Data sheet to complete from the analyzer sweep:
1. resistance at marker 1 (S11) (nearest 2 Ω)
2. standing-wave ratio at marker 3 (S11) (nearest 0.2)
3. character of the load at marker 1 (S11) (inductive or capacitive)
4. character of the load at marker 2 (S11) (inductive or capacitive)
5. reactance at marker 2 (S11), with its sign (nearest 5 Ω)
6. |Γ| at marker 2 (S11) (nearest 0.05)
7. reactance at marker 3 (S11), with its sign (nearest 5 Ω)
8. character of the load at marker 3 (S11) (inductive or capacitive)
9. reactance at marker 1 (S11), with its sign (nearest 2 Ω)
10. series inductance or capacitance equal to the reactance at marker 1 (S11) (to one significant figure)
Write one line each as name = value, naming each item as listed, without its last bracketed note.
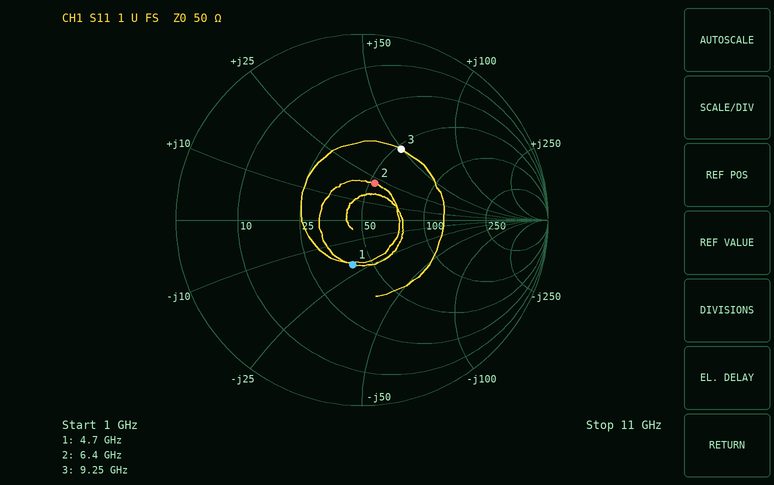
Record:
resistance at marker 1 (S11) = 40 Ω
standing-wave ratio at marker 3 (S11) = 2.6
character of the load at marker 1 (S11) = capacitive
character of the load at marker 2 (S11) = inductive
reactance at marker 2 (S11), with its sign = +20 Ω
|Γ| at marker 2 (S11) = 0.20
reactance at marker 3 (S11), with its sign = +50 Ω
character of the load at marker 3 (S11) = inductive
reactance at marker 1 (S11), with its sign = -20 Ω
series inductance or capacitance equal to the reactance at marker 1 (S11) = 2 pF
